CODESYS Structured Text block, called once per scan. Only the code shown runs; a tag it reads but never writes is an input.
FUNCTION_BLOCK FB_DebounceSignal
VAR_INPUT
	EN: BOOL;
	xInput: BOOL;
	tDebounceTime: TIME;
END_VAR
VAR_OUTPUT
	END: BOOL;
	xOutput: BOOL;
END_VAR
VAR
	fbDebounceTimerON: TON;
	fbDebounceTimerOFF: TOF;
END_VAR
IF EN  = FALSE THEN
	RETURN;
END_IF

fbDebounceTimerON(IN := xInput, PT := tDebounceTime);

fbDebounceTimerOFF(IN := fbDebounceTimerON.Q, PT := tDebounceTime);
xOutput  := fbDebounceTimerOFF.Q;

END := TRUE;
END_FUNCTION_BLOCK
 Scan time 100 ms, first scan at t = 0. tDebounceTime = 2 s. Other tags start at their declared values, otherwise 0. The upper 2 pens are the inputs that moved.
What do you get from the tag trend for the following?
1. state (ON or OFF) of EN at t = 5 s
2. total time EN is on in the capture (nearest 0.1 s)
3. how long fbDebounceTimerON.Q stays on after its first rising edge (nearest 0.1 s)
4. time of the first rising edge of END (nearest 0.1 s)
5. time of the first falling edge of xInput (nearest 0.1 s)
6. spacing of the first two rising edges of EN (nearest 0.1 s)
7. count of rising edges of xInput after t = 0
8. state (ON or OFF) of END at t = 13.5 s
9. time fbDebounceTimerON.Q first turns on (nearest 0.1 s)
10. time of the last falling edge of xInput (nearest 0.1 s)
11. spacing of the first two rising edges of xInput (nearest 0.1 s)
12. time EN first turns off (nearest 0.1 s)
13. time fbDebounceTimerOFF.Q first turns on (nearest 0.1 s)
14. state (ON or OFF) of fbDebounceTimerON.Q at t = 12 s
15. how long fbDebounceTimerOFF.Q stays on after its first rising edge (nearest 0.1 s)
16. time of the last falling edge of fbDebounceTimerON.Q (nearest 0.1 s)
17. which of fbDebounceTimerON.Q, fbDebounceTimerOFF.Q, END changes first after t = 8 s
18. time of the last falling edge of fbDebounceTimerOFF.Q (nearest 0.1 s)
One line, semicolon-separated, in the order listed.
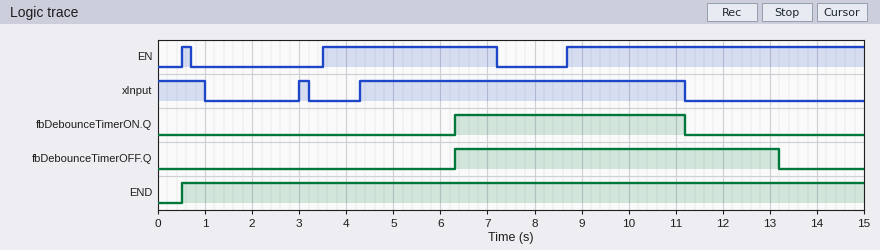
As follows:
ON; 10.2 s; 4.9 s; 0.5 s; 1.0 s; 3.0 s; 2; ON; 6.3 s; 11.2 s; 1.3 s; 0.7 s; 6.3 s; OFF; 6.9 s; 11.2 s; fbDebounceTimerON.Q; 13.2 s
